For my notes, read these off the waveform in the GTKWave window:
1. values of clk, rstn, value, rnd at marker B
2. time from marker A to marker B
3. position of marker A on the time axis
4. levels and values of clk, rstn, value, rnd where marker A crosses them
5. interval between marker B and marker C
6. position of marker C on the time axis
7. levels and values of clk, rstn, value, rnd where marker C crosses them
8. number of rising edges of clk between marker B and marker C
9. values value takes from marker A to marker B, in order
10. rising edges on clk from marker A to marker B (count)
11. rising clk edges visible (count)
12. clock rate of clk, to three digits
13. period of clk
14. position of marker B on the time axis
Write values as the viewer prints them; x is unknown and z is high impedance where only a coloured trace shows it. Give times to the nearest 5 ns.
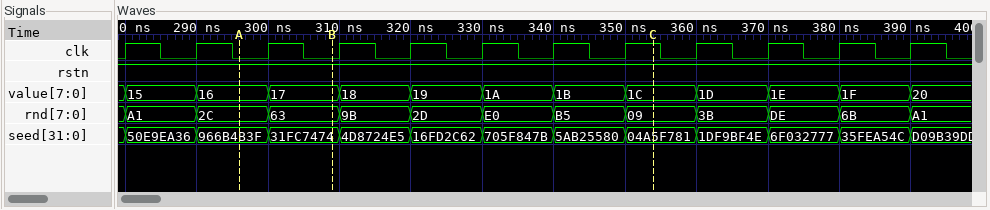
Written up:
clk=0, rstn=1, value=17, rnd=63
15 ns
295 ns
clk=0, rstn=1, value=16, rnd=2C
45 ns
355 ns
clk=1, rstn=1, value=1C, rnd=09
5
16, 17
1
12
100 MHz
10 ns
310 ns
